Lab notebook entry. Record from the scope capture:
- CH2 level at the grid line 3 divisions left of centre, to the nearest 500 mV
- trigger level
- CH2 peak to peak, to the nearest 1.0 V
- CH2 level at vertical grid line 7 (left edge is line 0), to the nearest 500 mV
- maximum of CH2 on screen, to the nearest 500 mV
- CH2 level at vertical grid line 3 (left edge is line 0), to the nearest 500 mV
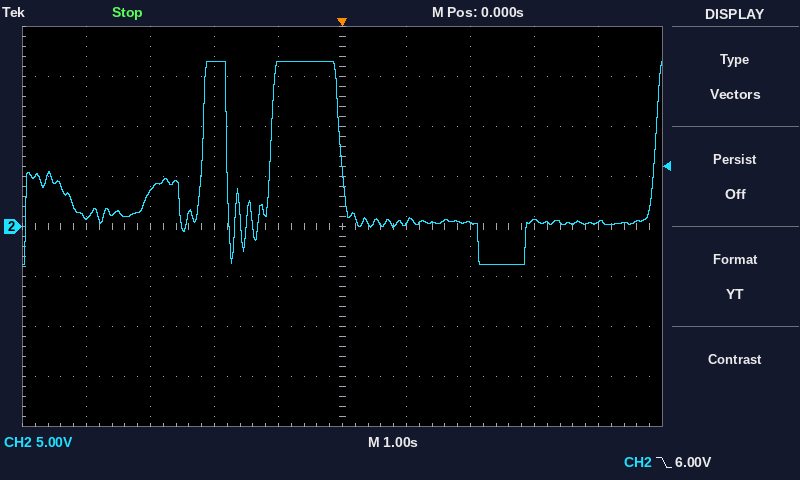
3.5 V
6.00 V
20.0 V
500 mV
16.5 V
16.5 V
